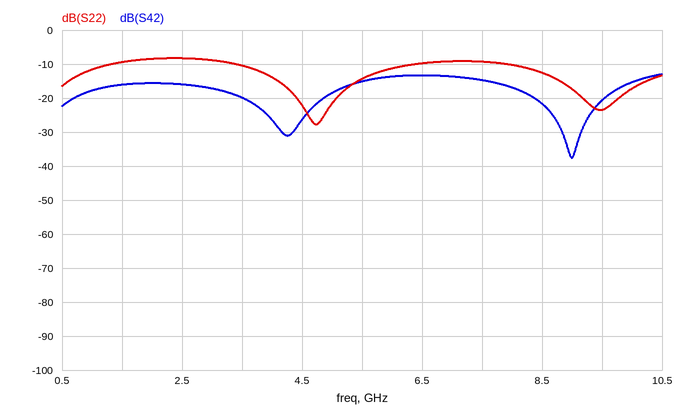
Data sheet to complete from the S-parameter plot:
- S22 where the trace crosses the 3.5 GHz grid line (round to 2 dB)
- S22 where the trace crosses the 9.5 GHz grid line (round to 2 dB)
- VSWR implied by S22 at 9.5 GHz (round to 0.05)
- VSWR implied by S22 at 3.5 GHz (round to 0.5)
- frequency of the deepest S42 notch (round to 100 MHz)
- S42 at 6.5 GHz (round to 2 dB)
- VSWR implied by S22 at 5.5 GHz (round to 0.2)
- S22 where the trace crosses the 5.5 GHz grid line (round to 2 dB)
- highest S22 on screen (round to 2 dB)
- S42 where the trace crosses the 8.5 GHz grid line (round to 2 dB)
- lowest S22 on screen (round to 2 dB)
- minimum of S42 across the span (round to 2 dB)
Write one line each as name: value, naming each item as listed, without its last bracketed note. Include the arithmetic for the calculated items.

S22 where the trace crosses the 3.5 GHz grid line: -10 dB
S22 where the trace crosses the 9.5 GHz grid line: -24 dB
VSWR implied by S22 at 9.5 GHz: |Γ| = 10^(-24/20) = 0.0631; VSWR = (1 + 0.0631)/(1 − 0.0631) ≈ 1.13, so 1.15 to the nearest 0.05
VSWR implied by S22 at 3.5 GHz: |Γ| = 10^(-10/20) = 0.3162; VSWR = (1 + 0.3162)/(1 − 0.3162) ≈ 1.92, so 2.0 to the nearest 0.5
frequency of the deepest S42 notch: 9.0 GHz
S42 at 6.5 GHz: -14 dB
VSWR implied by S22 at 5.5 GHz: |Γ| = 10^(-14/20) = 0.1995; VSWR = (1 + 0.1995)/(1 − 0.1995) ≈ 1.50, so 1.4 to the nearest 0.2
S22 where the trace crosses the 5.5 GHz grid line: -14 dB
highest S22 on screen: -8 dB
S42 where the trace crosses the 8.5 GHz grid line: -22 dB
lowest S22 on screen: -28 dB
minimum of S42 across the span: -38 dB
